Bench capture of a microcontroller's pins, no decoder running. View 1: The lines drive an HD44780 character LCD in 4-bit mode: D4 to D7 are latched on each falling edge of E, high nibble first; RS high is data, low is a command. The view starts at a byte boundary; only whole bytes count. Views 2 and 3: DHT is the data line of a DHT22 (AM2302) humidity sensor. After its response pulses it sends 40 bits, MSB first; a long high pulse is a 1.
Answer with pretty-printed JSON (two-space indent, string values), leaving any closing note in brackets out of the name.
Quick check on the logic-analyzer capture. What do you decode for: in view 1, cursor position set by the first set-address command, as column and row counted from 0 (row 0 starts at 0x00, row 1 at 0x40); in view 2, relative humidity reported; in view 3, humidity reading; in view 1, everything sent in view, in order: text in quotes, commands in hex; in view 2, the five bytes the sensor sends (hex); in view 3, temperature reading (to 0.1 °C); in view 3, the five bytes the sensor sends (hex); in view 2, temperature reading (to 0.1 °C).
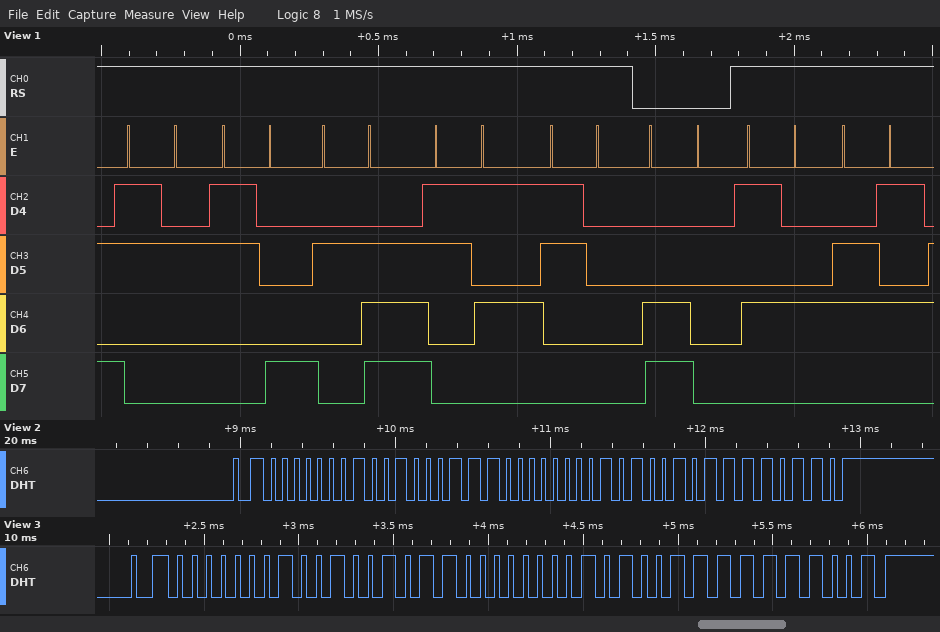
{
  "in view 1, cursor position set by the first set-address command, as column and row counted from 0": "column 0, row 1",
  "in view 2, relative humidity reported": "29.1 %",
  "in view 3, humidity reading": "29.3 %",
  "in view 1, everything sent in view, in order: text in quotes, commands in hex": "\"28.50\" 0xC0 \"Te\"",
  "in view 2, the five bytes the sensor sends": "01 23 80 52 F6",
  "in view 3, temperature reading": "-8.3 °C",
  "in view 3, the five bytes the sensor sends": "01 25 80 53 F9",
  "in view 2, temperature reading": "-8.2 °C"
}
